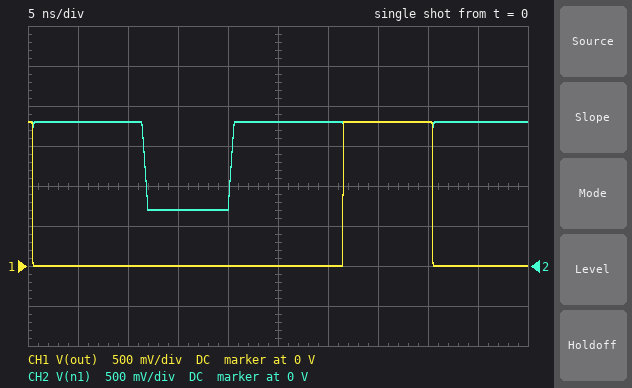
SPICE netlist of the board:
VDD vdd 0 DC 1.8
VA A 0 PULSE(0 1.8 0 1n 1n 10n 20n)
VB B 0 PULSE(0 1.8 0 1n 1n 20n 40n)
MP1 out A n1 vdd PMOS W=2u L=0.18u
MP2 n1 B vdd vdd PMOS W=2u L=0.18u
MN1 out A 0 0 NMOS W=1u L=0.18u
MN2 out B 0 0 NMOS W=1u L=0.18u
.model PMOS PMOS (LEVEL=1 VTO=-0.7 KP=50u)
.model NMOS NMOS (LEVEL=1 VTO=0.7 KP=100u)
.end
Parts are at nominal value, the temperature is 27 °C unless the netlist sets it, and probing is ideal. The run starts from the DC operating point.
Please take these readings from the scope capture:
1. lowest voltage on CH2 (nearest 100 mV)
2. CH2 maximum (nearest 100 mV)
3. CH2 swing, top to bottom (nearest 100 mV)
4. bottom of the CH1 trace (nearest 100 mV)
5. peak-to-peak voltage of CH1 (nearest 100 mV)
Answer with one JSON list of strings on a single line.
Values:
["700 mV", "1.8 V", "1.1 V", "0 V", "1.8 V"]
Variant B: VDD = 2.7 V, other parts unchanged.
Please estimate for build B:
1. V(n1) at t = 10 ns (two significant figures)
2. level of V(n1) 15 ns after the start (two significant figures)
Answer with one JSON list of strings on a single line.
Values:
["2.6 V", "900 mV"]
